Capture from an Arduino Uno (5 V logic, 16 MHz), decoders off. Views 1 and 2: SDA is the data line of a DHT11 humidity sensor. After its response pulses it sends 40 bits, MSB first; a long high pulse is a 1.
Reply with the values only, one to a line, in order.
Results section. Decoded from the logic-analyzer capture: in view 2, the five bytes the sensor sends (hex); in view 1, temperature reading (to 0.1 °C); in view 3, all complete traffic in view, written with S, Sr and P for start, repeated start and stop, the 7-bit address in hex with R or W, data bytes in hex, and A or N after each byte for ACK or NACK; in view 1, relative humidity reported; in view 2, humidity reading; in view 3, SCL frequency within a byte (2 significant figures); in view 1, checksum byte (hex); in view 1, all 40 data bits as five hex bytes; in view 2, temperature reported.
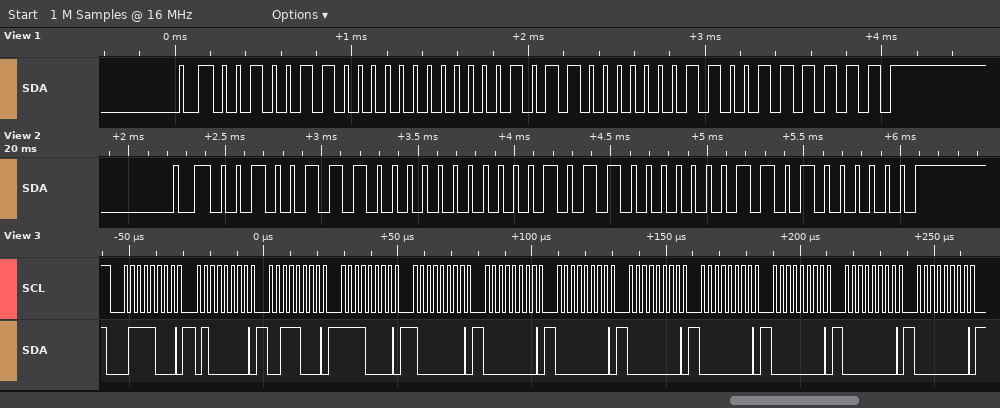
27 00 16 03 40
22.3 °C
S 3CW A 40 A 38 A F0 A 80 A 00 A 00 A 00 A 00 A 00 A 00 A 00 A
38 %
39 %
400 kHz
0x3F
26 00 16 03 3F
22.3 °C
